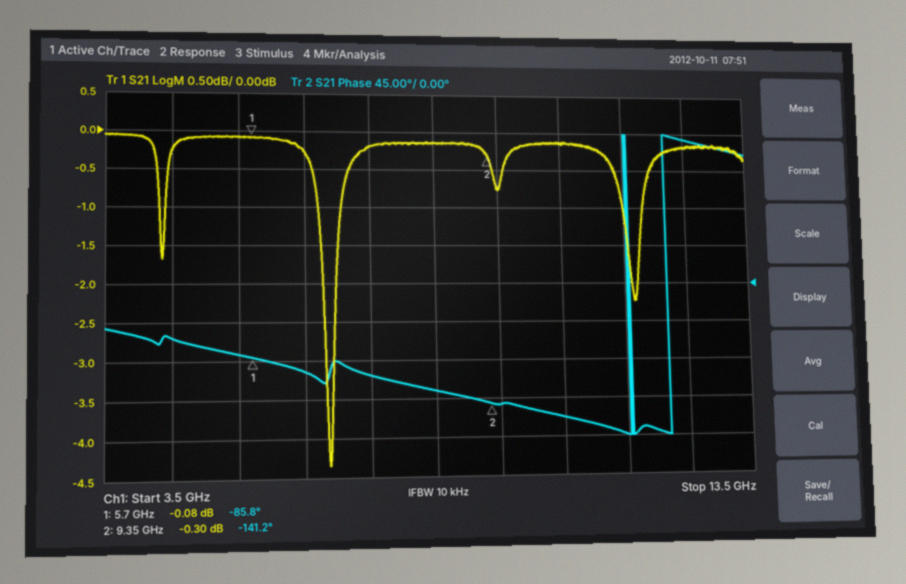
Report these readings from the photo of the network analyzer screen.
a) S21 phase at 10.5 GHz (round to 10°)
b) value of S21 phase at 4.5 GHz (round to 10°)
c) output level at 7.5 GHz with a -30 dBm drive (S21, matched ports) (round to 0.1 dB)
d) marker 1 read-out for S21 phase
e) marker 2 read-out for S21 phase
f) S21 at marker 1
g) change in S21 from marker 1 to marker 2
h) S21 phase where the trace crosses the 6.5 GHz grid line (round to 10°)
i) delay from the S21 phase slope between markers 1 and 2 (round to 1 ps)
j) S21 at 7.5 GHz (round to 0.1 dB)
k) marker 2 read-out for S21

-160°
-60°
-30.2 dBm
-85.8°
-141.2°
-0.08 dB
-0.22 dB
-100°
42 ps
-0.2 dB
-0.30 dB
